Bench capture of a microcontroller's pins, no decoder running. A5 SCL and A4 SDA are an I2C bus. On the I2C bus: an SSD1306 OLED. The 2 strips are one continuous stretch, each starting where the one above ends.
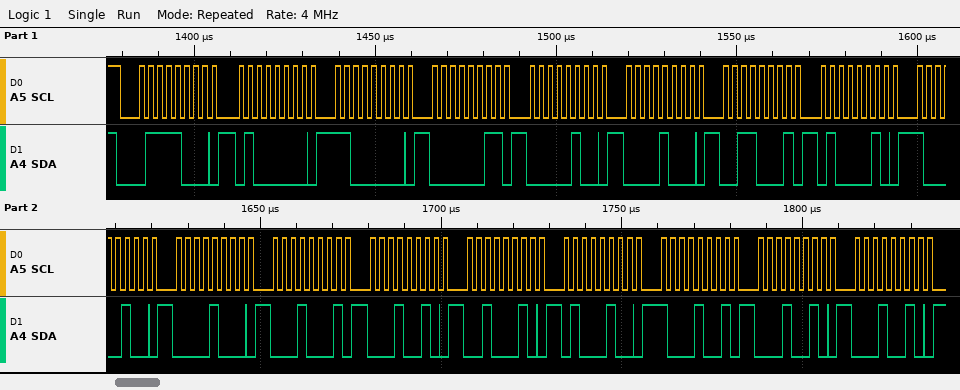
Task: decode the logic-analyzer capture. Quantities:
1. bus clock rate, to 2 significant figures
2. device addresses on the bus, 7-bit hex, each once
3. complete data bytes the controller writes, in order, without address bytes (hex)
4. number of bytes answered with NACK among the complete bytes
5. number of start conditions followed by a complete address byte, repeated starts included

400 kHz
0x3C
40 C0 03 04 08 31 42 84 08 11 12 22 44 89 12 12
0
1
